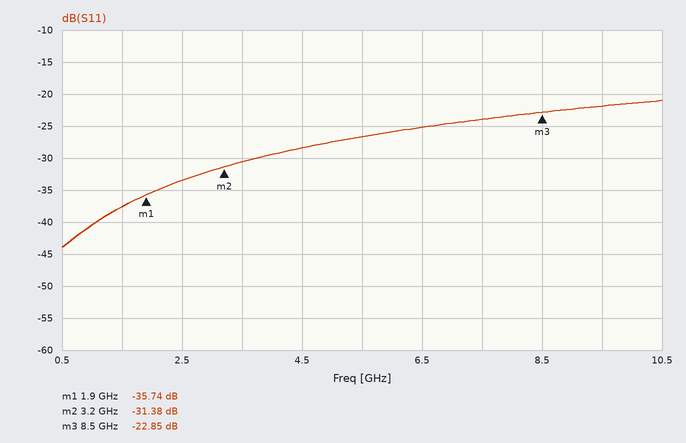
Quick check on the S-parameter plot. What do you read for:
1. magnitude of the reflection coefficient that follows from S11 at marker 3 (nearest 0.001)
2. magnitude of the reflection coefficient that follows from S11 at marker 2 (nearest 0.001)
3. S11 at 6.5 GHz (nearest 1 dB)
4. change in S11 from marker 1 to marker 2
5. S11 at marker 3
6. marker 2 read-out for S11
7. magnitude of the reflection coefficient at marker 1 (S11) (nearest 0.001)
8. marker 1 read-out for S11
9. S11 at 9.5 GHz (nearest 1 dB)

0.072
0.027
-25 dB
4.36 dB
-22.85 dB
-31.38 dB
0.016
-35.74 dB
-22 dB
